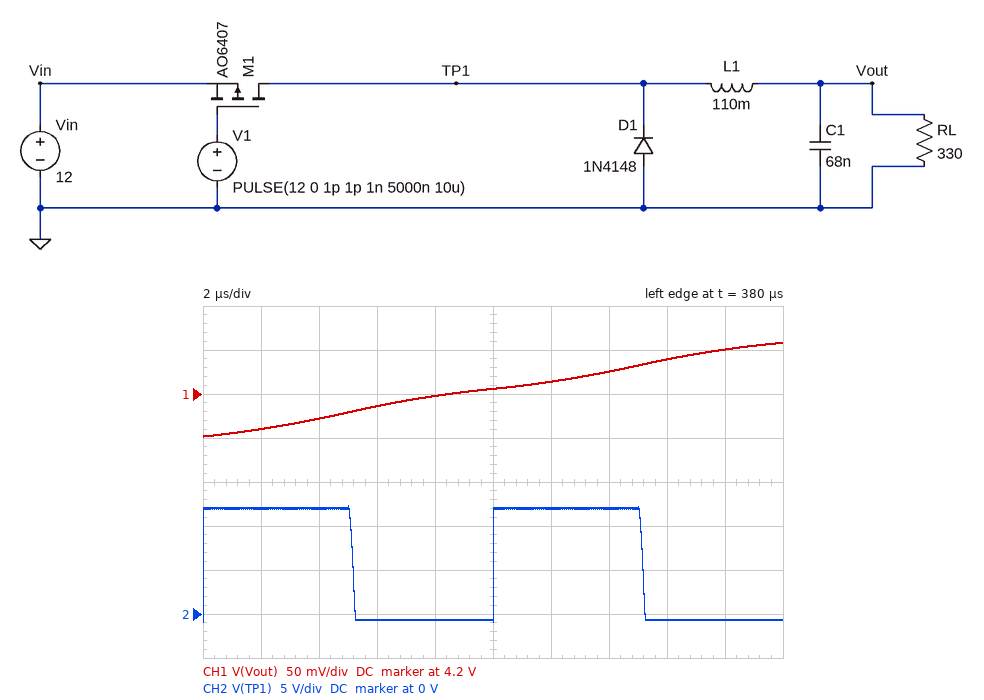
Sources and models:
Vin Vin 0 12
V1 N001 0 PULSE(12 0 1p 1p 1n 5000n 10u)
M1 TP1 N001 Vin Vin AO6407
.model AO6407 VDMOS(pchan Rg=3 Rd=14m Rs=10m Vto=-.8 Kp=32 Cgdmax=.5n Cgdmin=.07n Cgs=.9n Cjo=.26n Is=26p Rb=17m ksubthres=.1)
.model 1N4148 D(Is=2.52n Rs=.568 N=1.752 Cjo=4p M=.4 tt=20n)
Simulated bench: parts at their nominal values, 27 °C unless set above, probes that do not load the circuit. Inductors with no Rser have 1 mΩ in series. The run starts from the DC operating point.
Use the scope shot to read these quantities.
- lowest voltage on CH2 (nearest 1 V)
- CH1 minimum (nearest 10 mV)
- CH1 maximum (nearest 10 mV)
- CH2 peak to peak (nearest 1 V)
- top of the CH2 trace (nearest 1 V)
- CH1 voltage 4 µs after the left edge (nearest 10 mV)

-1 V
4.15 V
4.26 V
13 V
12 V
4.17 V
